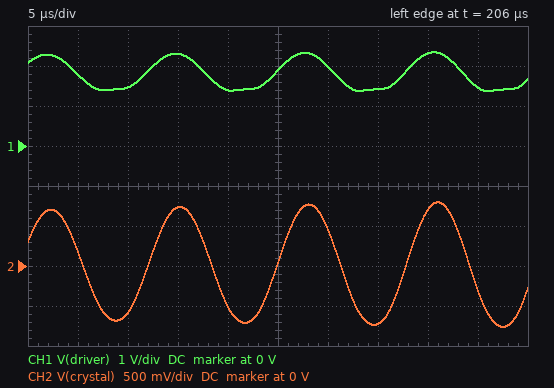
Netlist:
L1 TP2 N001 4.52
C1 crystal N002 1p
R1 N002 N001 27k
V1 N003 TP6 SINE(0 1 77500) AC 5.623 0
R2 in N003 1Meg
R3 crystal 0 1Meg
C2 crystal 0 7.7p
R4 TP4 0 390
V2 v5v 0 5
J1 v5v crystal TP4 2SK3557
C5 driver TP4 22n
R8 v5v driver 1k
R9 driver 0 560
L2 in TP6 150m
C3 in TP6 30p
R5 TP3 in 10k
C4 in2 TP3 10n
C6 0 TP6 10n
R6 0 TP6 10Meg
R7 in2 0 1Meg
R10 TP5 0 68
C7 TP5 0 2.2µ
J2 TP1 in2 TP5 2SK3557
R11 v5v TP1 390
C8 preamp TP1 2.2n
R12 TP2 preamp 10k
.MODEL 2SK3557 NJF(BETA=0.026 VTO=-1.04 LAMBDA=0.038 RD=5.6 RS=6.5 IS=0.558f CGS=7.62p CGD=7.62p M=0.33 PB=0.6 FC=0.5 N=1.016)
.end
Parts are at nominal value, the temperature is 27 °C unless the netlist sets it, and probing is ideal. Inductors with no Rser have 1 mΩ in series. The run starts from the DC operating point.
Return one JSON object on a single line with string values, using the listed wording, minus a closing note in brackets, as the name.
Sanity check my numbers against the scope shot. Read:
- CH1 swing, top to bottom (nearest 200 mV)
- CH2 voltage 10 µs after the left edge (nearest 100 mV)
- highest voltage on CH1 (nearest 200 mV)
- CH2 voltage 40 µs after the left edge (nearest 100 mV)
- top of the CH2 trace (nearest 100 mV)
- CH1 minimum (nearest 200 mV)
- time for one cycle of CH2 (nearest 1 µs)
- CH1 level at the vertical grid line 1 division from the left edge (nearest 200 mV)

{"CH1 swing, top to bottom": "1.0 V", "CH2 voltage 10 µs after the left edge": "-600 mV", "highest voltage on CH1": "2.4 V", "CH2 voltage 40 µs after the left edge": "700 mV", "top of the CH2 trace": "800 mV", "CH1 minimum": "1.4 V", "time for one cycle of CH2": "13 µs", "CH1 level at the vertical grid line 1 division from the left edge": "1.8 V"}
